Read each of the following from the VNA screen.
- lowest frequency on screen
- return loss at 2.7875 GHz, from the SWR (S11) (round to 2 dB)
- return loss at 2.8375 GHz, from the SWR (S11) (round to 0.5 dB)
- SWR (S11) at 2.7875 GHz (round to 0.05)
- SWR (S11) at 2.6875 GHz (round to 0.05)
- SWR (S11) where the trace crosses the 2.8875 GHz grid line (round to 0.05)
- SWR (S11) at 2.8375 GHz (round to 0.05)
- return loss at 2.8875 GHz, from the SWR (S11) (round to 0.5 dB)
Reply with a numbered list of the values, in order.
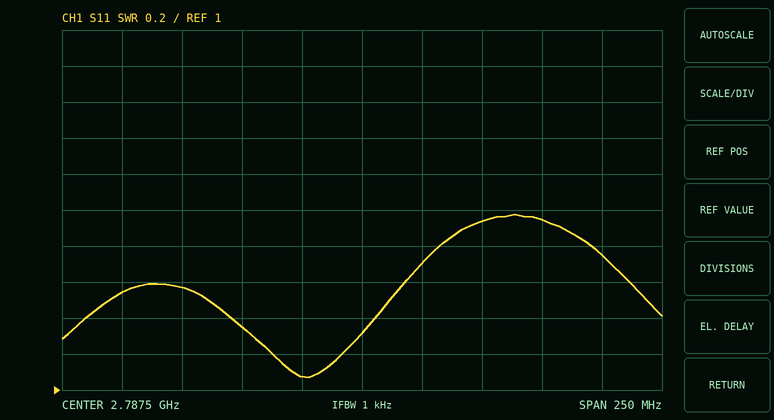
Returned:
1. 2.6625 GHz
2. 18 dB
3. 10.0 dB
4. 1.30
5. 1.55
6. 1.75
7. 1.95
8. 11.5 dB
